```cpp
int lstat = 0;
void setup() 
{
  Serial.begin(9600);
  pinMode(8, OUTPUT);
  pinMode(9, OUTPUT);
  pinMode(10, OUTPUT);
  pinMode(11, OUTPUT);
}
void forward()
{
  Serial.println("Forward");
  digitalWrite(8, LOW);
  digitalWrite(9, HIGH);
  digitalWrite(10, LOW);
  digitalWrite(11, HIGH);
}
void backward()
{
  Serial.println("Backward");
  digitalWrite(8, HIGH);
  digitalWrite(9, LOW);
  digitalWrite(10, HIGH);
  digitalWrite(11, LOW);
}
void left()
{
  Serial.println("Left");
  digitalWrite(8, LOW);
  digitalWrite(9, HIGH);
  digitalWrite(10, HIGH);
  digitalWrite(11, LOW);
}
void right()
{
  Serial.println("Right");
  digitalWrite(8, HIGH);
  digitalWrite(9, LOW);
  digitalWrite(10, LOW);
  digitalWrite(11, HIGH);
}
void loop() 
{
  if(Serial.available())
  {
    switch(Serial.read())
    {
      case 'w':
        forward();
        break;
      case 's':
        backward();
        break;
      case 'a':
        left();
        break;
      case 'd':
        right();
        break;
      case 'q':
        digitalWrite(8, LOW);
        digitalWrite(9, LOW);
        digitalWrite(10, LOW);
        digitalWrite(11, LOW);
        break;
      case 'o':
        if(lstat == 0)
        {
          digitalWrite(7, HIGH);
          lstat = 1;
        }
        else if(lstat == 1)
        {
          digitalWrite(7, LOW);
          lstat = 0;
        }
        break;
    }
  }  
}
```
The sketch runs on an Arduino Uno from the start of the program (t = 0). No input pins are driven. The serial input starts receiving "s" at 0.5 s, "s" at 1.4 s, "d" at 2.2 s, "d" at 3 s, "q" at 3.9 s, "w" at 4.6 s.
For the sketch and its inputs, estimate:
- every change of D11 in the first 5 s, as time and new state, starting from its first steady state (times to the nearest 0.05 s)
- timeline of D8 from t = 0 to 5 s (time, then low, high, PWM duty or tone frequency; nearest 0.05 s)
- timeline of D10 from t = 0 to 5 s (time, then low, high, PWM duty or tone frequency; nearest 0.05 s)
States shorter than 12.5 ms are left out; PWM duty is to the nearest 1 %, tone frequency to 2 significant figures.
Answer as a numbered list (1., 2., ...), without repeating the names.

1. 0 s low; 2.2 s high; 3.9 s low; 4.6 s high
2. 0 s low; 0.5 s high; 3.9 s low
3. 0 s low; 0.5 s high; 2.2 s low
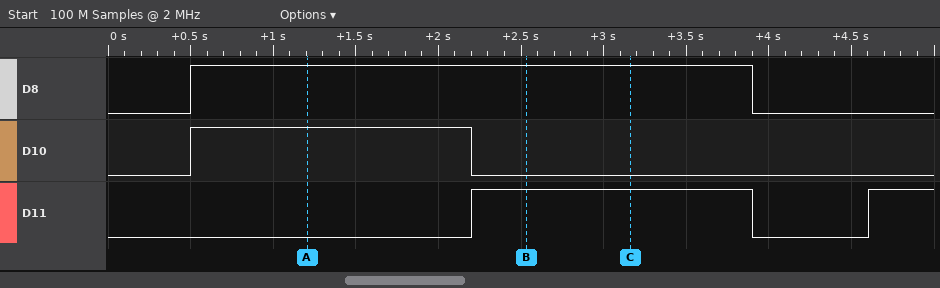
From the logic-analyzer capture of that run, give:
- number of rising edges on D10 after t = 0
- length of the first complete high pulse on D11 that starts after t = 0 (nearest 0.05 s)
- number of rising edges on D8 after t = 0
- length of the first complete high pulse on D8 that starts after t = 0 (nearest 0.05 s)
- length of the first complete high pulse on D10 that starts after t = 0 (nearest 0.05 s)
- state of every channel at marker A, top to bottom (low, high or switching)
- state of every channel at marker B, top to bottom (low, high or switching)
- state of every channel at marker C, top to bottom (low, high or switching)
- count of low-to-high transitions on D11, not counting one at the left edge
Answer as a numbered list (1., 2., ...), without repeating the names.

1. 1
2. 1.70 s
3. 1
4. 3.40 s
5. 1.70 s
6. D8 high, D10 high, D11 low
7. D8 high, D10 low, D11 high
8. D8 high, D10 low, D11 high
9. 2
